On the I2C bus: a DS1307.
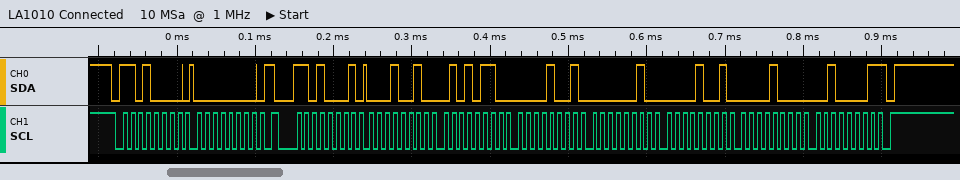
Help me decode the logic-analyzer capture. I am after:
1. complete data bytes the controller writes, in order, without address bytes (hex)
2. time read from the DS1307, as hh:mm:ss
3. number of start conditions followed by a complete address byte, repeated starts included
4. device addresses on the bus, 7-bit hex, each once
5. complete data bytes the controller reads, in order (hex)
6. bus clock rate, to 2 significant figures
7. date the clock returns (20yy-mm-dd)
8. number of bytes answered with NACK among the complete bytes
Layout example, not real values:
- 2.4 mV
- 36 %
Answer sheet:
- 00
- 09:56:12
- 2
- 0x68
- 12 56 09 02 09 08 21
- 100 kHz
- 2021-08-09
- 1
